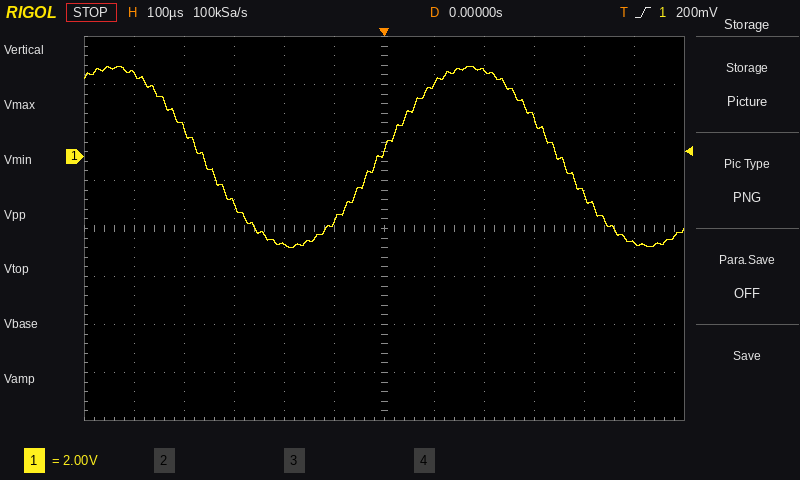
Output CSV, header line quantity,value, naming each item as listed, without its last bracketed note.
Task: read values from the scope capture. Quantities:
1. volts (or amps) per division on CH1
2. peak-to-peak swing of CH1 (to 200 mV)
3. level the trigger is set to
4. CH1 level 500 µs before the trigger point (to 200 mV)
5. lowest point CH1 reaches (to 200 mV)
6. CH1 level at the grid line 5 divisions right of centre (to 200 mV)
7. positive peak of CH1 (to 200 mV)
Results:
quantity,value
volts (or amps) per division on CH1,2 V
peak-to-peak swing of CH1,7.6 V
level the trigger is set to,200 mV
CH1 level 500 µs before the trigger point,3.4 V
lowest point CH1 reaches,-3.8 V
CH1 level at the grid line 5 divisions right of centre,-3.6 V
positive peak of CH1,3.8 V
